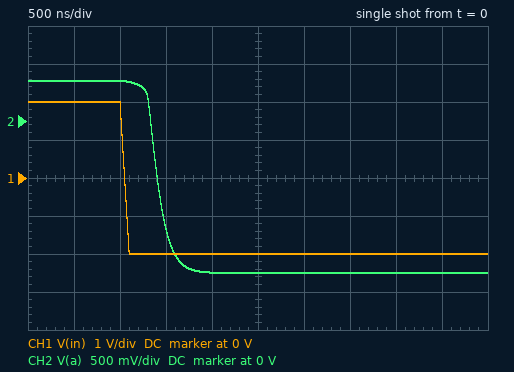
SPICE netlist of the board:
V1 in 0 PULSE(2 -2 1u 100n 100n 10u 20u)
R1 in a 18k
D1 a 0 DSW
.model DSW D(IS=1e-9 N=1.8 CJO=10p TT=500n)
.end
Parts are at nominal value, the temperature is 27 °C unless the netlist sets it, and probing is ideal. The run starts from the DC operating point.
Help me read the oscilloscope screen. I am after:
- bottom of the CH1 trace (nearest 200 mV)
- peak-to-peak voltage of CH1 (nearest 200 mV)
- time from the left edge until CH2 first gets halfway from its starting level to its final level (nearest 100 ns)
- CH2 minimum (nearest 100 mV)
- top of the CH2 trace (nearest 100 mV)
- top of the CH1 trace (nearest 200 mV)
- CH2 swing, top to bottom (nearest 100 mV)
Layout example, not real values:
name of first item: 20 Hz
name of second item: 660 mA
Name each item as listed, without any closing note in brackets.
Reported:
bottom of the CH1 trace: -2.0 V
peak-to-peak voltage of CH1: 4.0 V
time from the left edge until CH2 first gets halfway from its starting level to its final level: 1.4 µs
CH2 minimum: -2.0 V
top of the CH2 trace: 500 mV
top of the CH1 trace: 2.0 V
CH2 swing, top to bottom: 2.5 V
